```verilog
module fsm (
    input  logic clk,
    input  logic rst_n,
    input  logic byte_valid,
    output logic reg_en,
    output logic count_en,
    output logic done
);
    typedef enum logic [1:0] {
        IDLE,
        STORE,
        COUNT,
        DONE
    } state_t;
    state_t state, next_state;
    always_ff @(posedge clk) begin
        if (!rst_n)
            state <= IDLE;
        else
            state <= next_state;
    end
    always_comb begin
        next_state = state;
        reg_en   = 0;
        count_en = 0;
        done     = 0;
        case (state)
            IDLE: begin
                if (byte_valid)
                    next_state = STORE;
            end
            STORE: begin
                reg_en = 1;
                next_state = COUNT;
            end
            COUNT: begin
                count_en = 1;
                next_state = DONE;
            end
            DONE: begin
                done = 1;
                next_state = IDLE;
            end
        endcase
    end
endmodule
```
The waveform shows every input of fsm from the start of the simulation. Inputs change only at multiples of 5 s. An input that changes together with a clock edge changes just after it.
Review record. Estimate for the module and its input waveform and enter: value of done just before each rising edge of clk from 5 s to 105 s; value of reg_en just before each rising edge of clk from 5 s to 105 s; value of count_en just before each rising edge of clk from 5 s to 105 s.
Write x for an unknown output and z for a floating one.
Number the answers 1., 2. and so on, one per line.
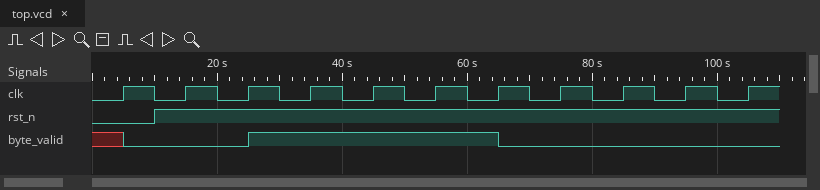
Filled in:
1. 0 0 0 0 0 0 1 0 0 0 0
2. 0 0 0 0 1 0 0 0 0 0 0
3. 0 0 0 0 0 1 0 0 0 0 0
